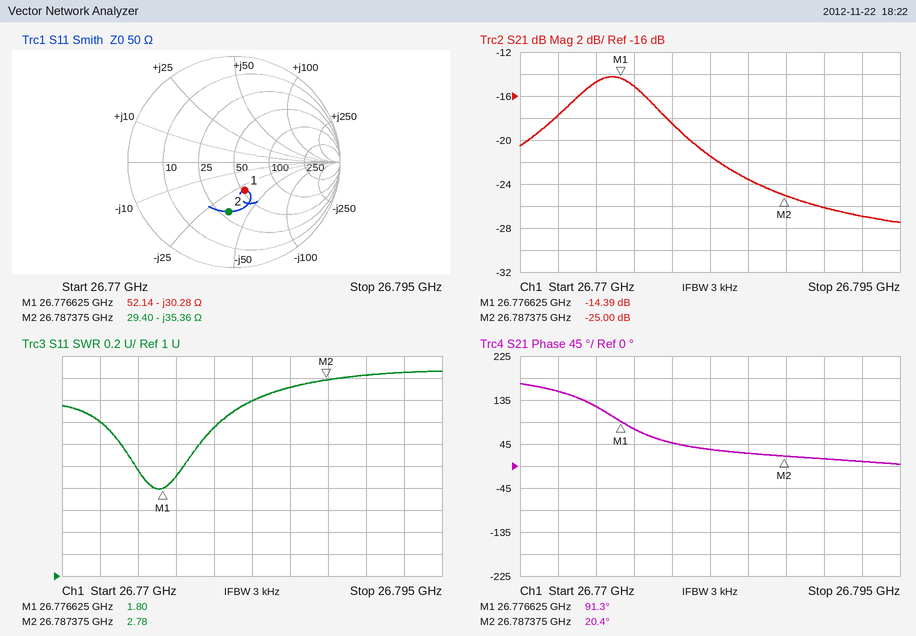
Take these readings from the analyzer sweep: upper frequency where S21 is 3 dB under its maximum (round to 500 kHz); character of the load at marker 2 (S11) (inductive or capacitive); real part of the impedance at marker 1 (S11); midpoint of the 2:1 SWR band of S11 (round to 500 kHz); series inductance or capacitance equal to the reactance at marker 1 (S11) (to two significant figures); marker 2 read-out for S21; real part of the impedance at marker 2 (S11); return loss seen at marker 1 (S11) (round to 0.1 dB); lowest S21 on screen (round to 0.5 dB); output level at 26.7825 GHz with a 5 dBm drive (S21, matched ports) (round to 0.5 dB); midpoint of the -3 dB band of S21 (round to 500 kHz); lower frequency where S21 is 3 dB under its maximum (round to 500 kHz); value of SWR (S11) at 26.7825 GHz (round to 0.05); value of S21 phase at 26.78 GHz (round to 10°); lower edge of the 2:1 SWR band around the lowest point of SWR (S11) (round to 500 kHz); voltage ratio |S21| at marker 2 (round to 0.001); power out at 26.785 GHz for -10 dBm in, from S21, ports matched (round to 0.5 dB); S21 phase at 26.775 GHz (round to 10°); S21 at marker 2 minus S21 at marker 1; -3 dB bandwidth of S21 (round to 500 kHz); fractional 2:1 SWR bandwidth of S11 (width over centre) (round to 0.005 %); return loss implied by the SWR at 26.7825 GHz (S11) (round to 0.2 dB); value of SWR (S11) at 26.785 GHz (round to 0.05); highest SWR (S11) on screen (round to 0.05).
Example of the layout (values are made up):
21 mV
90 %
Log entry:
26.7790 GHz
capacitive
52.14 Ω
26.7765 GHz
200 fF
-25.00 dB
29.40 Ω
10.9 dB
-27.5 dB
-16.5 dBm
26.7760 GHz
26.7730 GHz
2.60
50°
26.7750 GHz
0.056
-33.5 dBm
120°
-10.61 dB
6.0 MHz
0.010 %
7.0 dB
2.70
2.85
